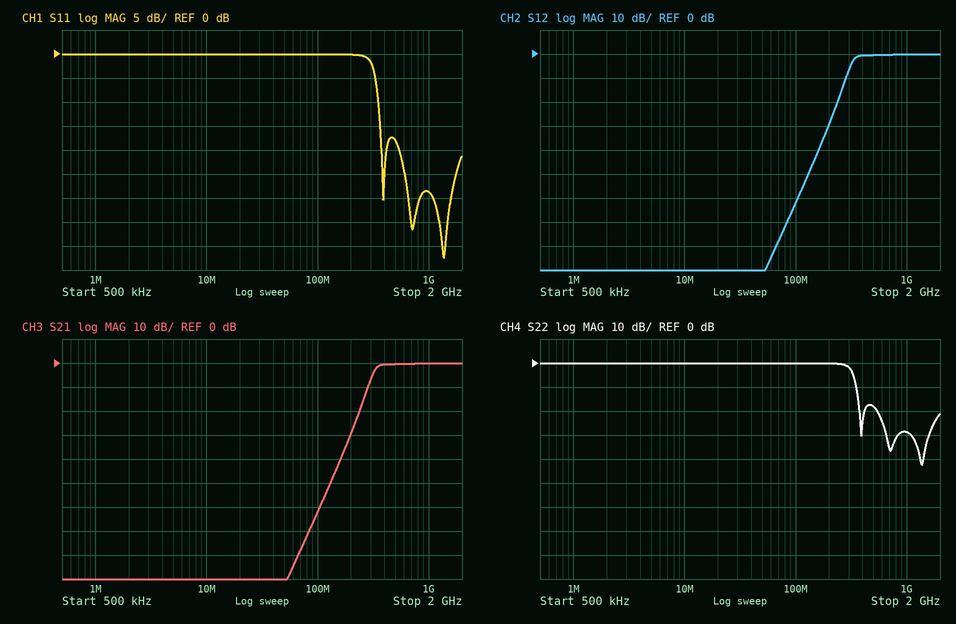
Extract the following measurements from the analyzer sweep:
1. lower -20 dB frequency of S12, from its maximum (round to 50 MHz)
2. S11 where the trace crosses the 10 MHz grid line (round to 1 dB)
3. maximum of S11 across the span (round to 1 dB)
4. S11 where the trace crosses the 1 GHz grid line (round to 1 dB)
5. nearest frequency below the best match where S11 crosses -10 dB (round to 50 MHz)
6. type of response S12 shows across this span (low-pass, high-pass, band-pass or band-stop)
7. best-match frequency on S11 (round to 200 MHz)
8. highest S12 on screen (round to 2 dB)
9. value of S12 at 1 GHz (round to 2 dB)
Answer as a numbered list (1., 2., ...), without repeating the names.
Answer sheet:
1. 250 MHz
2. 0 dB
3. 0 dB
4. -29 dB
5. 350 MHz
6. high-pass
7. 1.4 GHz
8. 0 dB
9. 0 dB
